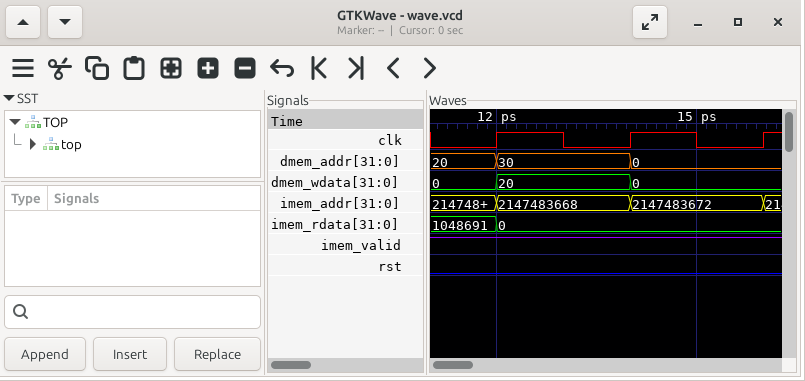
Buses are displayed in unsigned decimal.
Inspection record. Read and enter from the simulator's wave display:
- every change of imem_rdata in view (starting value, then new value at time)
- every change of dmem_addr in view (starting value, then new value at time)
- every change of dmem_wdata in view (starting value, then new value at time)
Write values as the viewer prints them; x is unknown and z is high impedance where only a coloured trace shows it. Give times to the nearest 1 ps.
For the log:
1048691, 0 at 12 ps
20, 30 at 12 ps, 0 at 14 ps
0, 20 at 12 ps, 0 at 14 ps
